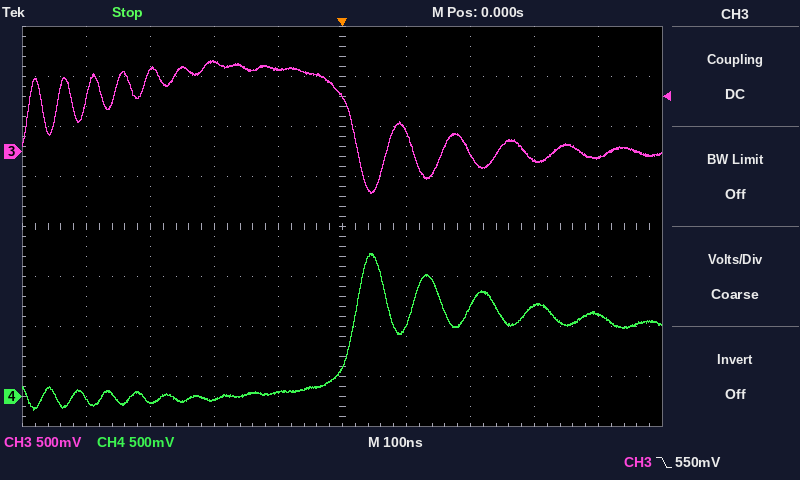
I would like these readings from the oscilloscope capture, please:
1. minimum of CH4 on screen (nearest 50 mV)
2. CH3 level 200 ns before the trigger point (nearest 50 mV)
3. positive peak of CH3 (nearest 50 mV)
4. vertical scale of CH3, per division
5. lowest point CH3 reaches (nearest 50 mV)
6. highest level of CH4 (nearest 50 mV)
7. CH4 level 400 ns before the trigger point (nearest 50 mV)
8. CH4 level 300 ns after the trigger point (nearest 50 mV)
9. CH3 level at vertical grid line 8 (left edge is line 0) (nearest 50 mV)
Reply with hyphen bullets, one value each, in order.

- -150 mV
- 900 mV
- 900 mV
- 500 mV
- -400 mV
- 1.45 V
- 0 mV
- 900 mV
- -100 mV
